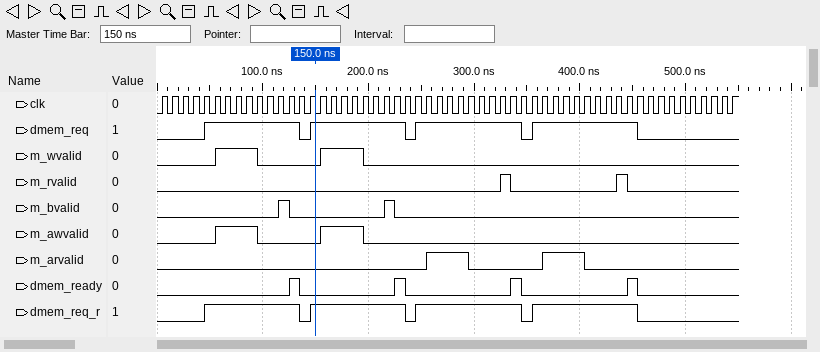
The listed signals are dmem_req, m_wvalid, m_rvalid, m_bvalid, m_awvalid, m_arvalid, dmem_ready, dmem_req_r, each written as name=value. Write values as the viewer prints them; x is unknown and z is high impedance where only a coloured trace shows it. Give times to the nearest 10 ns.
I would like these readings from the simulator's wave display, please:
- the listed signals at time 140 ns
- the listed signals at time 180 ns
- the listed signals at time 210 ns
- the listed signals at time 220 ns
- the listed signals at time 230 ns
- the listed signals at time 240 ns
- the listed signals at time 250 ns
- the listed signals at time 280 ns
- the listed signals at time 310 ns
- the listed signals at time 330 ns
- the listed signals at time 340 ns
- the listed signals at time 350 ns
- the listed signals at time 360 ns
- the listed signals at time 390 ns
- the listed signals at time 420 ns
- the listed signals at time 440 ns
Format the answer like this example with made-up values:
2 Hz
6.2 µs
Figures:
dmem_req=0, m_wvalid=0, m_rvalid=0, m_bvalid=0, m_awvalid=0, m_arvalid=0, dmem_ready=0, dmem_req_r=0
dmem_req=1, m_wvalid=1, m_rvalid=0, m_bvalid=0, m_awvalid=1, m_arvalid=0, dmem_ready=0, dmem_req_r=1
dmem_req=1, m_wvalid=0, m_rvalid=0, m_bvalid=0, m_awvalid=0, m_arvalid=0, dmem_ready=0, dmem_req_r=1
dmem_req=1, m_wvalid=0, m_rvalid=0, m_bvalid=1, m_awvalid=0, m_arvalid=0, dmem_ready=0, dmem_req_r=1
dmem_req=1, m_wvalid=0, m_rvalid=0, m_bvalid=0, m_awvalid=0, m_arvalid=0, dmem_ready=1, dmem_req_r=1
dmem_req=0, m_wvalid=0, m_rvalid=0, m_bvalid=0, m_awvalid=0, m_arvalid=0, dmem_ready=0, dmem_req_r=0
dmem_req=1, m_wvalid=0, m_rvalid=0, m_bvalid=0, m_awvalid=0, m_arvalid=0, dmem_ready=0, dmem_req_r=1
dmem_req=1, m_wvalid=0, m_rvalid=0, m_bvalid=0, m_awvalid=0, m_arvalid=1, dmem_ready=0, dmem_req_r=1
dmem_req=1, m_wvalid=0, m_rvalid=0, m_bvalid=0, m_awvalid=0, m_arvalid=0, dmem_ready=0, dmem_req_r=1
dmem_req=1, m_wvalid=0, m_rvalid=1, m_bvalid=0, m_awvalid=0, m_arvalid=0, dmem_ready=0, dmem_req_r=1
dmem_req=1, m_wvalid=0, m_rvalid=0, m_bvalid=0, m_awvalid=0, m_arvalid=0, dmem_ready=1, dmem_req_r=1
dmem_req=0, m_wvalid=0, m_rvalid=0, m_bvalid=0, m_awvalid=0, m_arvalid=0, dmem_ready=0, dmem_req_r=0
dmem_req=1, m_wvalid=0, m_rvalid=0, m_bvalid=0, m_awvalid=0, m_arvalid=0, dmem_ready=0, dmem_req_r=1
dmem_req=1, m_wvalid=0, m_rvalid=0, m_bvalid=0, m_awvalid=0, m_arvalid=1, dmem_ready=0, dmem_req_r=1
dmem_req=1, m_wvalid=0, m_rvalid=0, m_bvalid=0, m_awvalid=0, m_arvalid=0, dmem_ready=0, dmem_req_r=1
dmem_req=1, m_wvalid=0, m_rvalid=1, m_bvalid=0, m_awvalid=0, m_arvalid=0, dmem_ready=0, dmem_req_r=1
